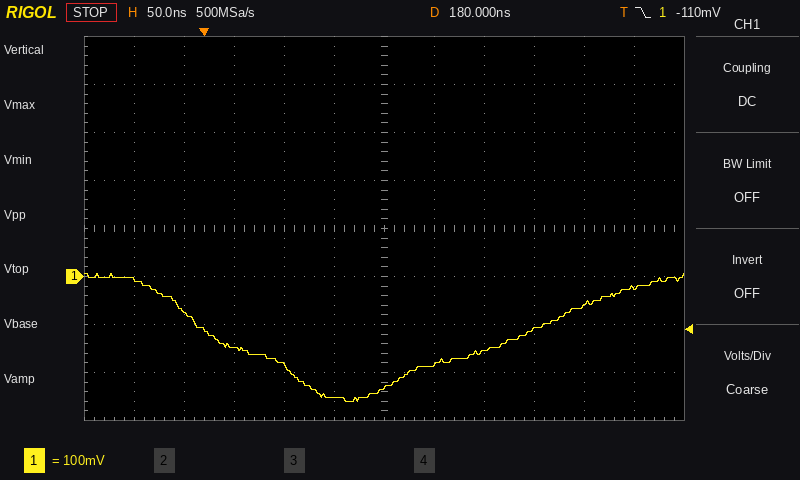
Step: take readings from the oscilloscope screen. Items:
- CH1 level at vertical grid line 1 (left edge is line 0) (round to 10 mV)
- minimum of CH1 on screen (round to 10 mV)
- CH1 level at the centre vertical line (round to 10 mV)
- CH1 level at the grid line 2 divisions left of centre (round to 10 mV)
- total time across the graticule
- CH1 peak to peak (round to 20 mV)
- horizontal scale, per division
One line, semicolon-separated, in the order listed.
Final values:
-10 mV; -260 mV; -230 mV; -190 mV; 600 ns; 260 mV; 50 ns
